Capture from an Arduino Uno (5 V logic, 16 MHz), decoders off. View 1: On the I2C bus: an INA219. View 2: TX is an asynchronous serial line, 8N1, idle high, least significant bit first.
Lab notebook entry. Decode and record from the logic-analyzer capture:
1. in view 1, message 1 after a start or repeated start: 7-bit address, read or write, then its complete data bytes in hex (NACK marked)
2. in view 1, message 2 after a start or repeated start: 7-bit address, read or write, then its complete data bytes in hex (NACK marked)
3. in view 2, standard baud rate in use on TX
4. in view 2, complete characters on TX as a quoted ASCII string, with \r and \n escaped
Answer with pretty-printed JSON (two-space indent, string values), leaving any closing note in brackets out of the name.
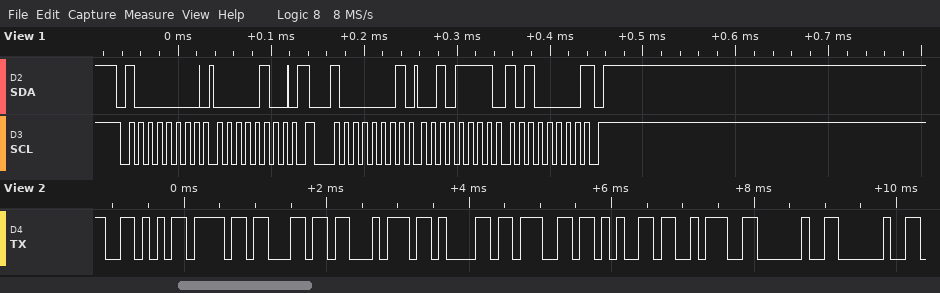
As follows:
{
  "in view 1, message 1 after a start or repeated start: 7-bit address, read or write, then its complete data bytes in hex": "0x40 write: 04",
  "in view 1, message 2 after a start or repeated start: 7-bit address, read or write, then its complete data bytes in hex": "0x40 read: 2F A0 NACK",
  "in view 2, standard baud rate in use on TX": "9600 baud",
  "in view 2, complete characters on TX as a quoted ASCII string, with \\r and \\n escaped": "\"Voltage:  \""
}
